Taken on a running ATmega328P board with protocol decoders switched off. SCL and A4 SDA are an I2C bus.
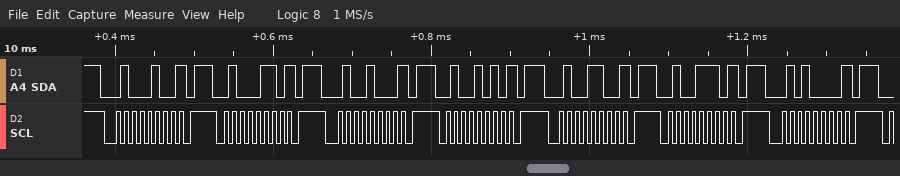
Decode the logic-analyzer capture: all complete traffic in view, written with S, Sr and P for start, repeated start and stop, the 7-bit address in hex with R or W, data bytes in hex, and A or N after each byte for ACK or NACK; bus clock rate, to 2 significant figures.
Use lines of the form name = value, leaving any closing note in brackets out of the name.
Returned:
all complete traffic in view, written with S, Sr and P for start, repeated start and stop, the 7-bit address in hex with R or W, data bytes in hex, and A or N after each byte for ACK or NACK = S 22W N P S 23W N P S 24W N P S 25W N P S 26W N P S 27W N P S 28W N P
bus clock rate, to 2 significant figures = 100 kHz
